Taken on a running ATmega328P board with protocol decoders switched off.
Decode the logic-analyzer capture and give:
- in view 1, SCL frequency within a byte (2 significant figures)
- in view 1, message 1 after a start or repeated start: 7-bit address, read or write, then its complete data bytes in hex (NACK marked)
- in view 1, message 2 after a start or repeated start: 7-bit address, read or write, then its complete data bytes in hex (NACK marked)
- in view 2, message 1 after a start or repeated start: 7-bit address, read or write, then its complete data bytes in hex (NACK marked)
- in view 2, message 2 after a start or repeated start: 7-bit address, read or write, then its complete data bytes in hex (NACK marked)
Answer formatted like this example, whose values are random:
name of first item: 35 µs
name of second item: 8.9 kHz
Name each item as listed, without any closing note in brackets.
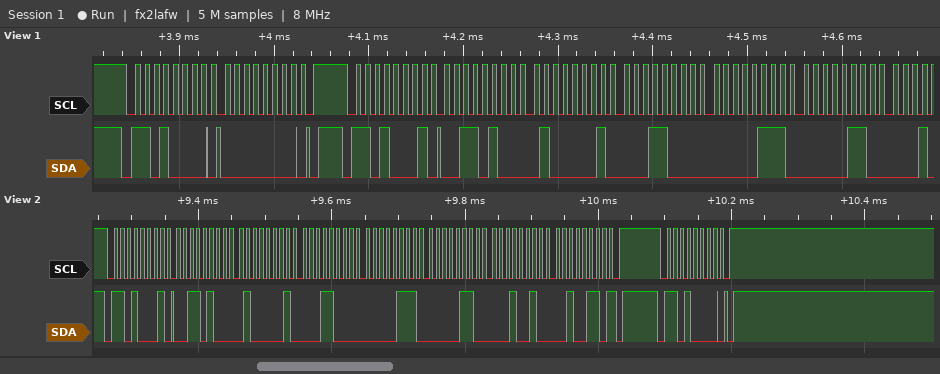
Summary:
in view 1, SCL frequency within a byte: 100 kHz
in view 1, message 1 after a start or repeated start: 7-bit address, read or write, then its complete data bytes in hex: 0x68 write: 00
in view 1, message 2 after a start or repeated start: 7-bit address, read or write, then its complete data bytes in hex: 0x68 read: 34 41 18 07 06
in view 2, message 1 after a start or repeated start: 7-bit address, read or write, then its complete data bytes in hex: 0x68 read: 34 41 18 07 06 12 26 NACK
in view 2, message 2 after a start or repeated start: 7-bit address, read or write, then its complete data bytes in hex: 0x68 write
